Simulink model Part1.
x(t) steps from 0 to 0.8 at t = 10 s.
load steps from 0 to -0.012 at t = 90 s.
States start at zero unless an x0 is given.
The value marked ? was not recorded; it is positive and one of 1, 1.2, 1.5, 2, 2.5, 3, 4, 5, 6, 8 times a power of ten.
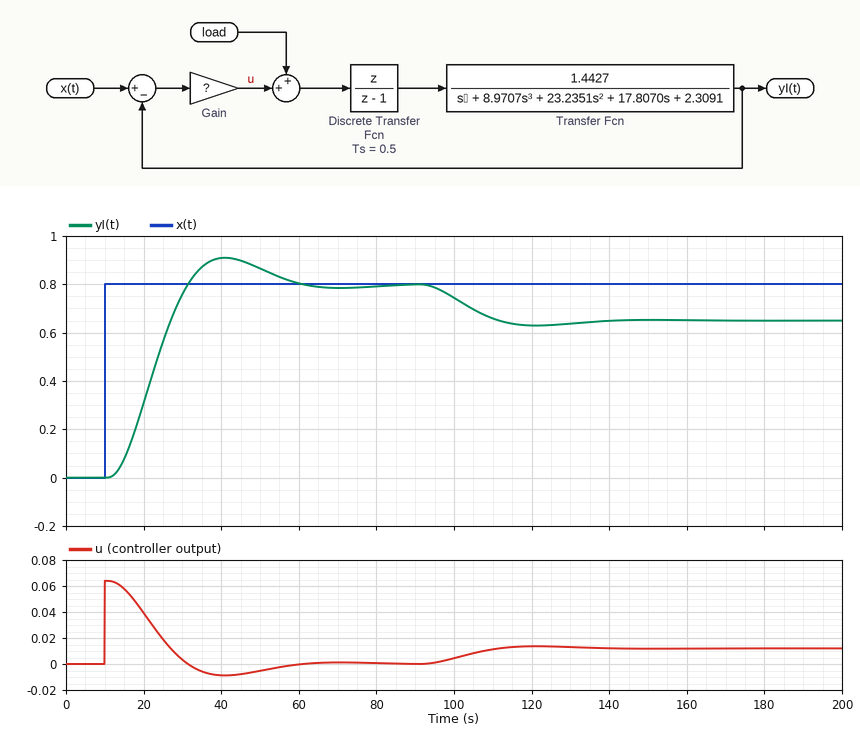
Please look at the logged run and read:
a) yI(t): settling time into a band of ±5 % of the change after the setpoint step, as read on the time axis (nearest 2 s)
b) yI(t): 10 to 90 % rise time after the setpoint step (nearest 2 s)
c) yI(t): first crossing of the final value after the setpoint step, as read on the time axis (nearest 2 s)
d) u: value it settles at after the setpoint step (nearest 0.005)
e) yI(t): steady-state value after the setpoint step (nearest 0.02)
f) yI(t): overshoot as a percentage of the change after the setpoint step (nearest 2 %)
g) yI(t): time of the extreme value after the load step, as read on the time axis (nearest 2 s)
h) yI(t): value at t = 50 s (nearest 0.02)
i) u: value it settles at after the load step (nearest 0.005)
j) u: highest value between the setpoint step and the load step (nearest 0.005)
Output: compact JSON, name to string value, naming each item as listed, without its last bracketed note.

{"yI(t): settling time into a band of ±5 % of the change after the setpoint step, as read on the time axis": "54 s", "yI(t): 10 to 90 % rise time after the setpoint step": "14 s", "yI(t): first crossing of the final value after the setpoint step, as read on the time axis": "32 s", "u: value it settles at after the setpoint step": "0.000", "yI(t): steady-state value after the setpoint step": "0.80", "yI(t): overshoot as a percentage of the change after the setpoint step": "14 %", "yI(t): time of the extreme value after the load step, as read on the time axis": "122 s", "yI(t): value at t = 50 s": "0.86", "u: value it settles at after the load step": "0.010", "u: highest value between the setpoint step and the load step": "0.065"}
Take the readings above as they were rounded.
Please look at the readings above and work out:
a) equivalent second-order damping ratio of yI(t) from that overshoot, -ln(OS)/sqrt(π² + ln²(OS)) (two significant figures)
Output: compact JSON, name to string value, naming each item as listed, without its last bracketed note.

{"equivalent second-order damping ratio of yI(t) from that overshoot, -ln(OS)/sqrt(π² + ln²(OS))": "0.53"}
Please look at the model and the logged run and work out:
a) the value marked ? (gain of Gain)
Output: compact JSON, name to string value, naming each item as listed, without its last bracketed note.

{"the value marked ?": "0.08"}
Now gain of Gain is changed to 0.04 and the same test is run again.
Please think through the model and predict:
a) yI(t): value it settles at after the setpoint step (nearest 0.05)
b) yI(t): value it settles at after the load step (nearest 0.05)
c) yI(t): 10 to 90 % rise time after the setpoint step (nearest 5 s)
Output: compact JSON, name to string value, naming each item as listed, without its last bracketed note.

{"yI(t): value it settles at after the setpoint step": "0.80", "yI(t): value it settles at after the load step": "0.50", "yI(t): 10 to 90 % rise time after the setpoint step": "30 s"}
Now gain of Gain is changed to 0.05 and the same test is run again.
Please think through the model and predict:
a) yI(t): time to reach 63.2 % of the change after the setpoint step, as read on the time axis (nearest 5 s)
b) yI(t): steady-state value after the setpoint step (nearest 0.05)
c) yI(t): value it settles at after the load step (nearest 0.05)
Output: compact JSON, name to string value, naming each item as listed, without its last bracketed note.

{"yI(t): time to reach 63.2 % of the change after the setpoint step, as read on the time axis": "30 s", "yI(t): steady-state value after the setpoint step": "0.80", "yI(t): value it settles at after the load step": "0.55"}
